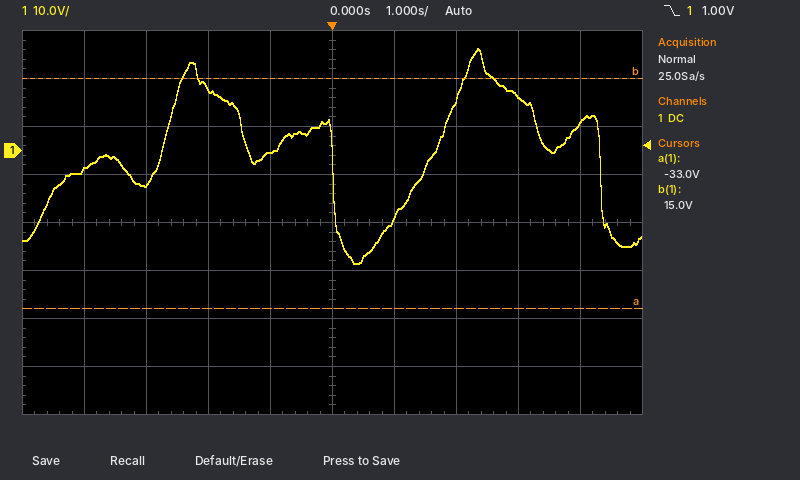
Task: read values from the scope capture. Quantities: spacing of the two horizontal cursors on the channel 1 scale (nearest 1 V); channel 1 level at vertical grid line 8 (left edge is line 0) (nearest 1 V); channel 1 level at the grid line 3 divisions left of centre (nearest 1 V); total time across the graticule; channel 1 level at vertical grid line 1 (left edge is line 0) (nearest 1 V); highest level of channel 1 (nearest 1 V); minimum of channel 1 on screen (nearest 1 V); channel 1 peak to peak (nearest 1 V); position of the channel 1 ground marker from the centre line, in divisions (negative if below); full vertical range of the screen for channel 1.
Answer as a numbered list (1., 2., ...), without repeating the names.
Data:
1. 48 V
2. 11 V
3. -7 V
4. 10 s
5. -4 V
6. 21 V
7. -24 V
8. 45 V
9. +1.5 div
10. 80 V
